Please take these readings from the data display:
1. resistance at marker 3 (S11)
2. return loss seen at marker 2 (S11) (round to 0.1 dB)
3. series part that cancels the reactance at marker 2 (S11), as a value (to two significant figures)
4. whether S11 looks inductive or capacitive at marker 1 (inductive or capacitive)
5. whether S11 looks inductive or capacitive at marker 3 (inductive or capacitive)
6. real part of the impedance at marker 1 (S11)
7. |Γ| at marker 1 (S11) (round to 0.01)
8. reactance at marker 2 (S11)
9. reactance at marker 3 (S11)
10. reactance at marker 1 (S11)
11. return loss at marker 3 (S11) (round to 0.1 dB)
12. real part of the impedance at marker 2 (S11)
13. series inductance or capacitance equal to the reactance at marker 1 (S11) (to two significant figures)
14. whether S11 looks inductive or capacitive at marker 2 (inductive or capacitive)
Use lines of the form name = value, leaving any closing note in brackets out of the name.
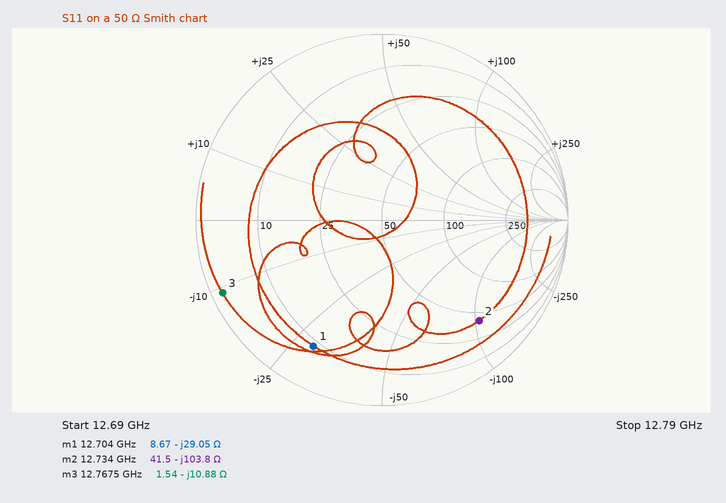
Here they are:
resistance at marker 3 = 1.54 Ω
return loss seen at marker 2 (S11) = 2.5 dB
series part that cancels the reactance at marker 2 (S11), as a value = 1.3 nH
whether S11 looks inductive or capacitive at marker 1 = capacitive
whether S11 looks inductive or capacitive at marker 3 = capacitive
real part of the impedance at marker 1 = 8.67 Ω
|Γ| at marker 1 (S11) = 0.77
reactance at marker 2 = -103.8 Ω
reactance at marker 3 = -10.88 Ω
reactance at marker 1 = -29.05 Ω
return loss at marker 3 (S11) = 0.5 dB
real part of the impedance at marker 2 = 41.5 Ω
series inductance or capacitance equal to the reactance at marker 1 (S11) = 430 fF
whether S11 looks inductive or capacitive at marker 2 = capacitive
